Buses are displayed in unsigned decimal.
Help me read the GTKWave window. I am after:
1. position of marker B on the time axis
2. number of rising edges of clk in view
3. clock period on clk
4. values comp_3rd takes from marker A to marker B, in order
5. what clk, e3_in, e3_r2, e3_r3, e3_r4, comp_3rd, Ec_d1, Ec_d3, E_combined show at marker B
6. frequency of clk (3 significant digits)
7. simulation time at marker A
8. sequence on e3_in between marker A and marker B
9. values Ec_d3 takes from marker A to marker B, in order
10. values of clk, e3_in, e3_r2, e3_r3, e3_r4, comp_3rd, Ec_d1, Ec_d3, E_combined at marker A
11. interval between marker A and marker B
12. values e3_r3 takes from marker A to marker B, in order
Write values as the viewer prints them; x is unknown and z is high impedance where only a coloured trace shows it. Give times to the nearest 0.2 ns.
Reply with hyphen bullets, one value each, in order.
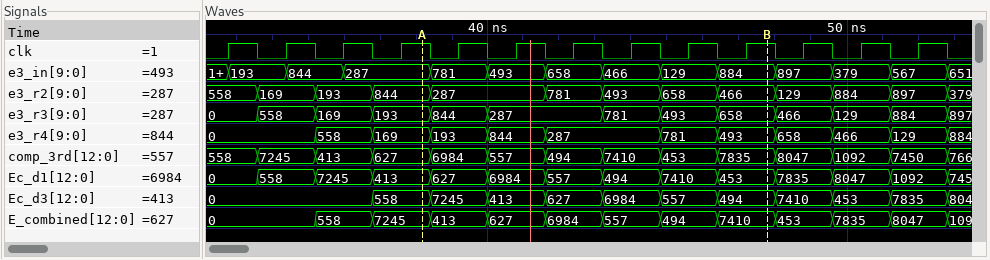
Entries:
- 47.8 ns
- 13
- 1.6 ns
- 627, 6984, 557, 494, 7410, 453, 7835
- clk=1, e3_in=884, e3_r2=466, e3_r3=658, e3_r4=493, comp_3rd=7835, Ec_d1=453, Ec_d3=494, E_combined=7410
- 625 MHz
- 38.2 ns
- 287, 781, 493, 658, 466, 129, 884
- 558, 7245, 413, 627, 6984, 557, 494
- clk=1, e3_in=287, e3_r2=844, e3_r3=193, e3_r4=169, comp_3rd=627, Ec_d1=413, Ec_d3=558, E_combined=7245
- 9.6 ns
- 193, 844, 287, 781, 493, 658
